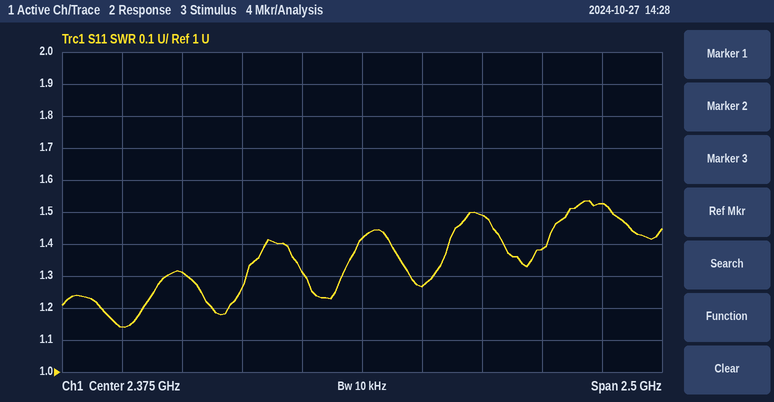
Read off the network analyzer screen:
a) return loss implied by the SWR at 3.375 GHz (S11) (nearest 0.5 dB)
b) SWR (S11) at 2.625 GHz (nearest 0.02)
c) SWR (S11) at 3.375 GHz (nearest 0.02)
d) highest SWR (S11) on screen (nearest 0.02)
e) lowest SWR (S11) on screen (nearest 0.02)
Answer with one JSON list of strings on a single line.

["13.5 dB", "1.26", "1.52", "1.54", "1.14"]
